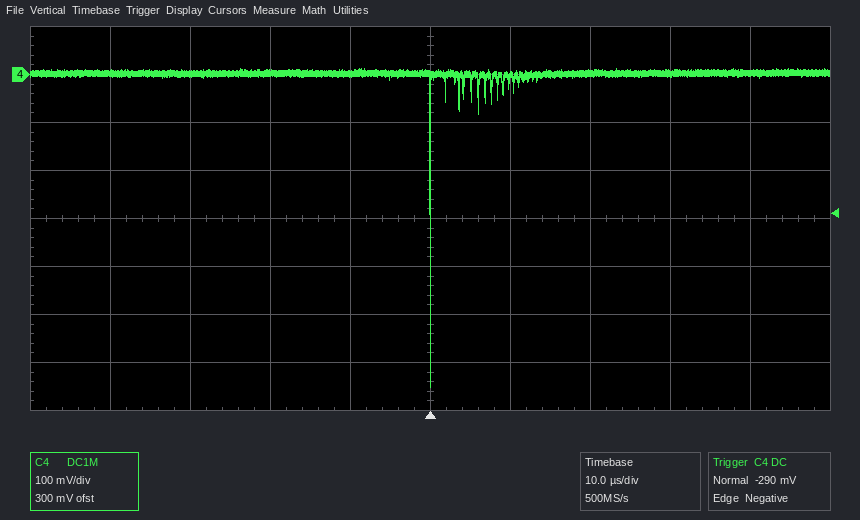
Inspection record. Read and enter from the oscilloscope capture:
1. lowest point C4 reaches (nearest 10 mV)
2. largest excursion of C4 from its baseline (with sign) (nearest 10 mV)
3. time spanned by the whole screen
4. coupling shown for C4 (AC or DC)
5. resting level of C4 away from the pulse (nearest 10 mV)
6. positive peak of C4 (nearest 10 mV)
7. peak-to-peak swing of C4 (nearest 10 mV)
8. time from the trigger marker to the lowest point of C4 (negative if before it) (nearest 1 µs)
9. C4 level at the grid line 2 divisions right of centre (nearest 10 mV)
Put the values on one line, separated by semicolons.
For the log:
-650 mV; -650 mV; 100 µs; DC; 0 mV; 10 mV; 660 mV; 0 µs; 0 mV
